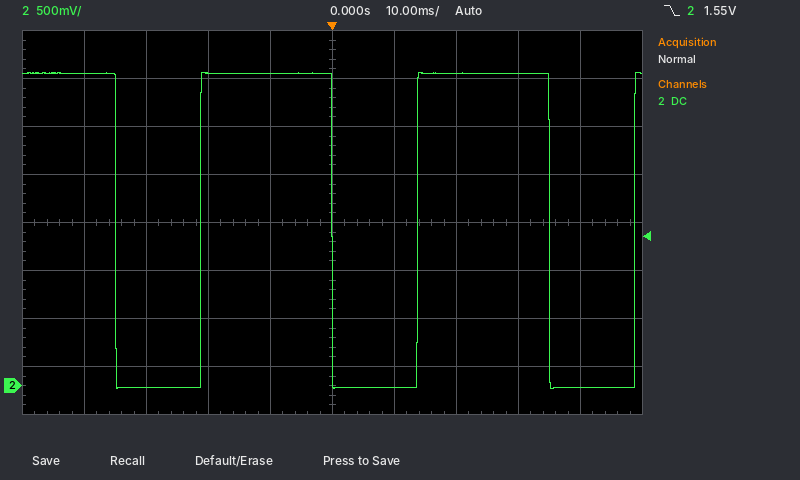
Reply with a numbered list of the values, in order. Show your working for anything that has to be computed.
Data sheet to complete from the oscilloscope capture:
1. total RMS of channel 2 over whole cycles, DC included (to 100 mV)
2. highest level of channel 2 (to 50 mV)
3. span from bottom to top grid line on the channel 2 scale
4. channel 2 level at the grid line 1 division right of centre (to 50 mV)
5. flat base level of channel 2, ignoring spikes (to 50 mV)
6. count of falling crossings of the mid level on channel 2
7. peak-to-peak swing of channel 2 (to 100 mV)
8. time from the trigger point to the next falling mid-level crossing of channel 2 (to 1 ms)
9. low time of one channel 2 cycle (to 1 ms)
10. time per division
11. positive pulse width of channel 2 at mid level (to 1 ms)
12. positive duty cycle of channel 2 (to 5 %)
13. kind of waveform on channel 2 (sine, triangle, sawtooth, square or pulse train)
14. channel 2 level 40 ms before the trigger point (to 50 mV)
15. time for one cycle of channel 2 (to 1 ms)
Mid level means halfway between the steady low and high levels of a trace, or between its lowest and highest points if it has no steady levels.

1. √(0.6 × (3.25 V)² + 0.4 × (0 mV)²) ≈ 2.5 V
2. 3.25 V
3. 4 V
4. 0 mV
5. 0 mV
6. 3
7. 3.30 V
8. 35 ms
9. 14 ms
10. 10 ms
11. 21 ms
12. 21 ms / 35 ms ≈ 60 %
13. pulse train
14. 3.25 V
15. 35 ms
